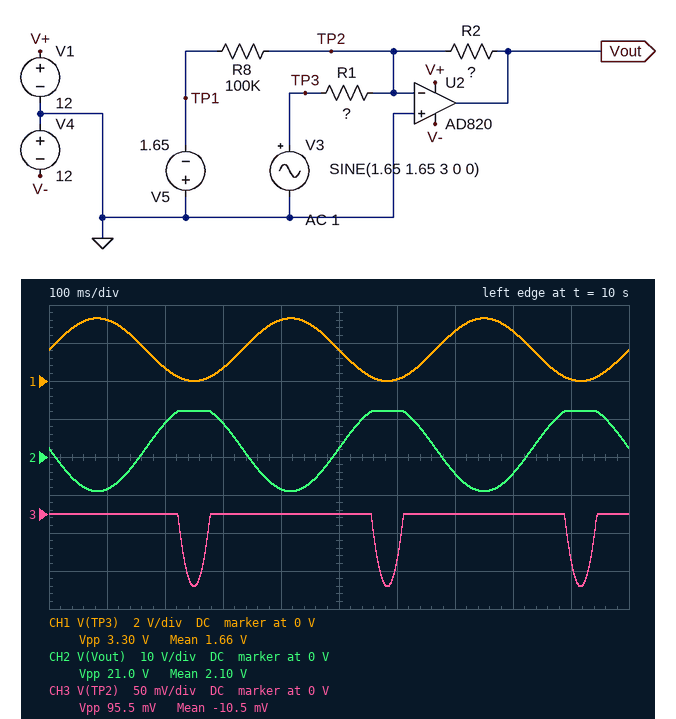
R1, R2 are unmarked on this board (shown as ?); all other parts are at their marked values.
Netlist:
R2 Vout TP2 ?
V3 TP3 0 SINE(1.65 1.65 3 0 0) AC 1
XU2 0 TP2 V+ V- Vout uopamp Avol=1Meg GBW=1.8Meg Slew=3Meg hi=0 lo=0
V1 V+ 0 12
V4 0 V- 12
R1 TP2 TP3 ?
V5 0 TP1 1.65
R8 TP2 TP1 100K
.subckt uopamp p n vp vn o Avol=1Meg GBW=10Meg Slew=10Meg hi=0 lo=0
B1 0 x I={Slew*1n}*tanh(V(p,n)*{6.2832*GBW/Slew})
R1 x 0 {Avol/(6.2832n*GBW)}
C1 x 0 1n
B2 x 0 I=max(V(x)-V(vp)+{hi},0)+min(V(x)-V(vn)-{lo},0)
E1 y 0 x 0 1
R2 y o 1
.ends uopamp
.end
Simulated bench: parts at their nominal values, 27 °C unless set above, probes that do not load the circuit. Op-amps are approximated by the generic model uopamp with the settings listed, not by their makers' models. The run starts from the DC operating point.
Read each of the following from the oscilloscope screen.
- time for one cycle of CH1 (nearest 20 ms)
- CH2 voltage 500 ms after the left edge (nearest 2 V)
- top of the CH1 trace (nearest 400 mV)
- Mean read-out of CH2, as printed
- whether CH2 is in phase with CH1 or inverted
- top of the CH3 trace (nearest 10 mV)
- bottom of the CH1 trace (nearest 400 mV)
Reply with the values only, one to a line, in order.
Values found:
340 ms
2 V
3.2 V
2.10 V
inverted
0 V
0 V
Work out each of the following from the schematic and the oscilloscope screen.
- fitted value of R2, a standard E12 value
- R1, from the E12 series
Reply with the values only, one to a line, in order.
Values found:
820 kΩ
120 kΩ
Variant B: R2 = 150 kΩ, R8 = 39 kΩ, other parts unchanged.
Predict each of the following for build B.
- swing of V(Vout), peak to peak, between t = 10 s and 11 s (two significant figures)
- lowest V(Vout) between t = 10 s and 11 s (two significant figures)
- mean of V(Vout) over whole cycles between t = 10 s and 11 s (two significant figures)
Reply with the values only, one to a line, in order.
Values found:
4.1 V
2.2 V
4.3 V
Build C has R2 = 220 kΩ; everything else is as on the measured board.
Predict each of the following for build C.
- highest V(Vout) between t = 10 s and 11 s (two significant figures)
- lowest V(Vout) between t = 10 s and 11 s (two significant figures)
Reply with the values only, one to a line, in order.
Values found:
3.6 V
-2.4 V
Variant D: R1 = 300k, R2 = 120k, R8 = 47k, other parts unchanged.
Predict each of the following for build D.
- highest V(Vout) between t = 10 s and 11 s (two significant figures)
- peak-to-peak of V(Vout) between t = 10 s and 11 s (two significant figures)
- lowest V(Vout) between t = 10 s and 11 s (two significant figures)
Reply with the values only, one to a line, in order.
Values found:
4.2 V
1.3 V
2.9 V
